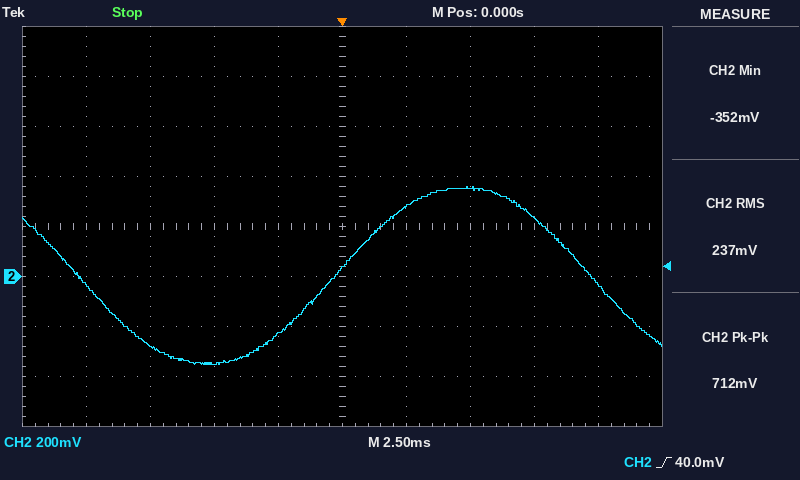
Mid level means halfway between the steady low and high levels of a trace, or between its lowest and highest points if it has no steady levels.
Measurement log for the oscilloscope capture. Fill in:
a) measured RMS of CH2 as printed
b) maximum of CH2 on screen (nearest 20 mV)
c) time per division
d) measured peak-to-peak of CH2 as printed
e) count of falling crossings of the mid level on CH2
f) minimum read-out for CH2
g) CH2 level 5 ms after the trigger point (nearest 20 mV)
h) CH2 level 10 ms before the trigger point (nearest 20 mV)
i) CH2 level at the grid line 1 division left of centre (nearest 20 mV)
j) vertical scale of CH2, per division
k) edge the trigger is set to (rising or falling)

237 mV
360 mV
2.5 ms
712 mV
2
-352 mV
360 mV
-40 mV
-240 mV
200 mV
rising
